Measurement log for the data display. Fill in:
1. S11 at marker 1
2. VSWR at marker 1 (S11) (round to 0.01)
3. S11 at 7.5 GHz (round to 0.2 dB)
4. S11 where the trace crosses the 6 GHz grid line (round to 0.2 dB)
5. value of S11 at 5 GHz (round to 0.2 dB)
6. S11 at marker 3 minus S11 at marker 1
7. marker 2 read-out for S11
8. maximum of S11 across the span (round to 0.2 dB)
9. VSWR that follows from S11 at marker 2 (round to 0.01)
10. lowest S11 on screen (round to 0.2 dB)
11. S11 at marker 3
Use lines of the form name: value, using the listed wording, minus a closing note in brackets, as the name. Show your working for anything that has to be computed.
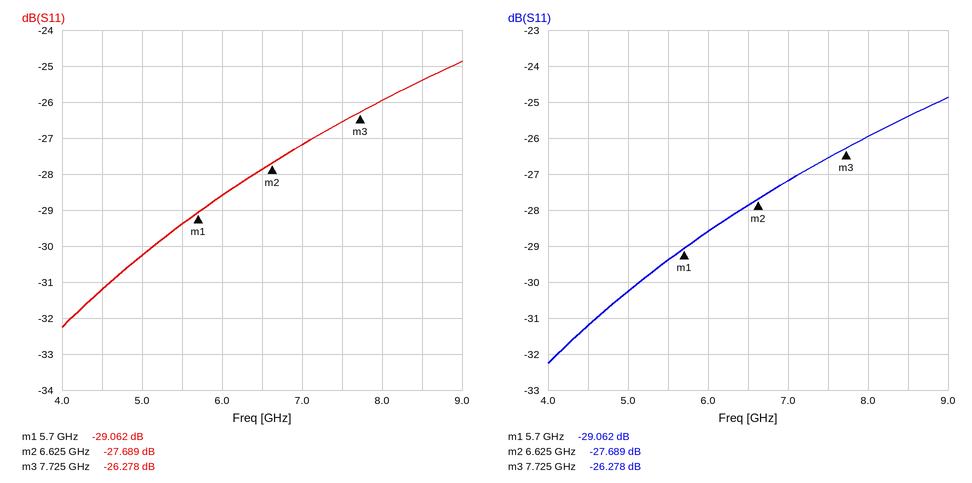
S11 at marker 1: -29.062 dB
VSWR at marker 1 (S11): (1 + 0.0352)/(1 − 0.0352) ≈ 1.07
S11 at 7.5 GHz: -26.6 dB
S11 where the trace crosses the 6 GHz grid line: -28.6 dB
value of S11 at 5 GHz: -30.2 dB
S11 at marker 3 minus S11 at marker 1: -26.278 − (-29.062) = 2.784 dB
marker 2 read-out for S11: -27.689 dB
maximum of S11 across the span: -24.8 dB
VSWR that follows from S11 at marker 2: (1 + 0.0413)/(1 − 0.0413) ≈ 1.09
lowest S11 on screen: -32.2 dB
S11 at marker 3: -26.278 dB
